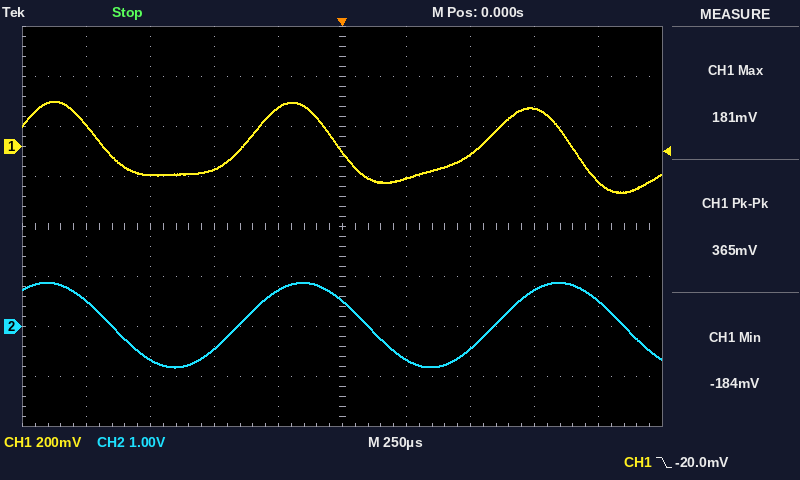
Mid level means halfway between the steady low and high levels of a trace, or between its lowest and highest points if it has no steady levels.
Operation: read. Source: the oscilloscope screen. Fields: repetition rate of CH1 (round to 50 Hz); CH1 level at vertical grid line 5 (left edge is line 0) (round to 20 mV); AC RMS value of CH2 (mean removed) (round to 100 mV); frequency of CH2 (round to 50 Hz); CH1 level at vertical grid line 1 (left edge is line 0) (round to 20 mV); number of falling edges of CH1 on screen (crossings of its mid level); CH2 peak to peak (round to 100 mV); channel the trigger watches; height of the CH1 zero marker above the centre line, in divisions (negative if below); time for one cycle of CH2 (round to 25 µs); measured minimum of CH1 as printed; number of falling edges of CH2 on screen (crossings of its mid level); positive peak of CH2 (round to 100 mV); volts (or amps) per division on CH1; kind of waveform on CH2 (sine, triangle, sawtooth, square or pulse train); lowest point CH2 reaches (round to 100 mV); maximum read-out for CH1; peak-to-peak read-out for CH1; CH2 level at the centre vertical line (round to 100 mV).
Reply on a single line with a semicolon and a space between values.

1.10 kHz; -20 mV; 600 mV; 1.00 kHz; 80 mV; 3; 1.7 V; CH1; +1.6 div; 1.000 ms; -184 mV; 3; 900 mV; 200 mV; sine; -800 mV; 181 mV; 365 mV; 500 mV
